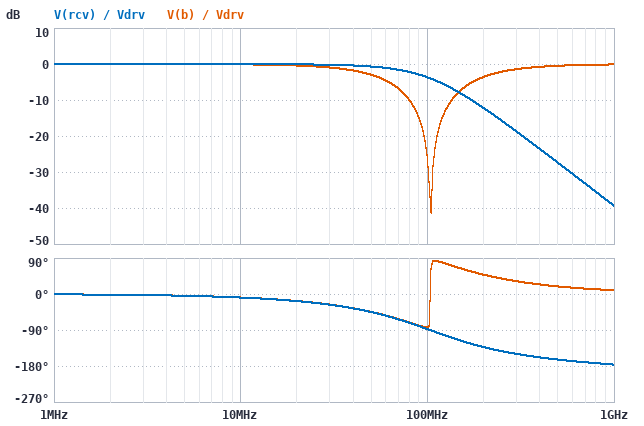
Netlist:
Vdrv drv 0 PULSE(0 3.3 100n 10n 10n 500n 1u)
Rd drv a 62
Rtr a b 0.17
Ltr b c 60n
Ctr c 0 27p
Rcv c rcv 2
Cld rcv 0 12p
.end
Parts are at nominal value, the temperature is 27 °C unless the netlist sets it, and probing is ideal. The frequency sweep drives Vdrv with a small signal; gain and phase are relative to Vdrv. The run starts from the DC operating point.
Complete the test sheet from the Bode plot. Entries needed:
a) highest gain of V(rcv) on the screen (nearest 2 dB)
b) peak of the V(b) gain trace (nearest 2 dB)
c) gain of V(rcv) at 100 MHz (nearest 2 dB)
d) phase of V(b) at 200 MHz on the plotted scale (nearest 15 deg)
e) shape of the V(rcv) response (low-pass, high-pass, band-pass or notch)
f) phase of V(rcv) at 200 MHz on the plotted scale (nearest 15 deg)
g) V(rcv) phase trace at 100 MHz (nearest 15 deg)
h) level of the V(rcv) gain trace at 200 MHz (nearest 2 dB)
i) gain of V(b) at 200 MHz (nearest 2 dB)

0 dB
0 dB
-4 dB
45 deg
low-pass
-135 deg
-90 deg
-12 dB
-4 dB
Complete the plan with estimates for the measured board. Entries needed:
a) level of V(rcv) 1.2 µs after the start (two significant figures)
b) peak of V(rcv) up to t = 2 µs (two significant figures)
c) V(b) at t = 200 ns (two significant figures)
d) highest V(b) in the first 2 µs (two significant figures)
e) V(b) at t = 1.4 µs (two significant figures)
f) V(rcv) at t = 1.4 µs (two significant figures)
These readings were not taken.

3.3 V
3.3 V
3.3 V
3.3 V
3.3 V
3.3 V
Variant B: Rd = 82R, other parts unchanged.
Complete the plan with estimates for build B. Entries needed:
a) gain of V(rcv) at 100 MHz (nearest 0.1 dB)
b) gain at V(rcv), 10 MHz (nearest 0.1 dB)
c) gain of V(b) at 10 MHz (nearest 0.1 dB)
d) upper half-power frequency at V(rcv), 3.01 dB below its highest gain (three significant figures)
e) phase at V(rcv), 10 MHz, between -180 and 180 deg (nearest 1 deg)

-6.1 dB
-0.1 dB
-0.2 dB
62.5 MHz
-12 deg
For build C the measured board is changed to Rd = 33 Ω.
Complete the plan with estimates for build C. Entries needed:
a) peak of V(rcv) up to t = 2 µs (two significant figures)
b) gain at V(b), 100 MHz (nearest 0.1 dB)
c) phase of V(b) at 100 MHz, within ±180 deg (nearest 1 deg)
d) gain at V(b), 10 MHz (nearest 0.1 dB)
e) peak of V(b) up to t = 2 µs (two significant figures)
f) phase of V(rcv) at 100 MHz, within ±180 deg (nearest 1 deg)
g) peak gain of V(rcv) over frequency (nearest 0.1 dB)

3.5 V
-20.6 dB
-81 deg
0 dB
3.4 V
-85 deg
2.3 dB
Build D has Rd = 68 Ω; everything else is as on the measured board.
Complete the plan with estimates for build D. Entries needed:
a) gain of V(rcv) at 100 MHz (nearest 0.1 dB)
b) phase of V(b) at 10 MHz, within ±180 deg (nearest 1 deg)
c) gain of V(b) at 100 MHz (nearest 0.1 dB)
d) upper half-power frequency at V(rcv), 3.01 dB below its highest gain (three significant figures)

-4.5 dB
-10 deg
-26.8 dB
81.1 MHz
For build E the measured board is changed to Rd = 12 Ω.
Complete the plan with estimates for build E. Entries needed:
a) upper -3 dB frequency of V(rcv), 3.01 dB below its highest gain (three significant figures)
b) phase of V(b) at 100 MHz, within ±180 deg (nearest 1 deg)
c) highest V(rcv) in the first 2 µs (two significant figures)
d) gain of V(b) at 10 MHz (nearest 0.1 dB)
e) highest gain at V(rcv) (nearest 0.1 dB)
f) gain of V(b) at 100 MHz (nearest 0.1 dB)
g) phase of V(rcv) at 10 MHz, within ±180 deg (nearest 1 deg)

117 MHz
-72 deg
3.5 V
0 dB
10.1 dB
-12.2 dB
-2 deg
